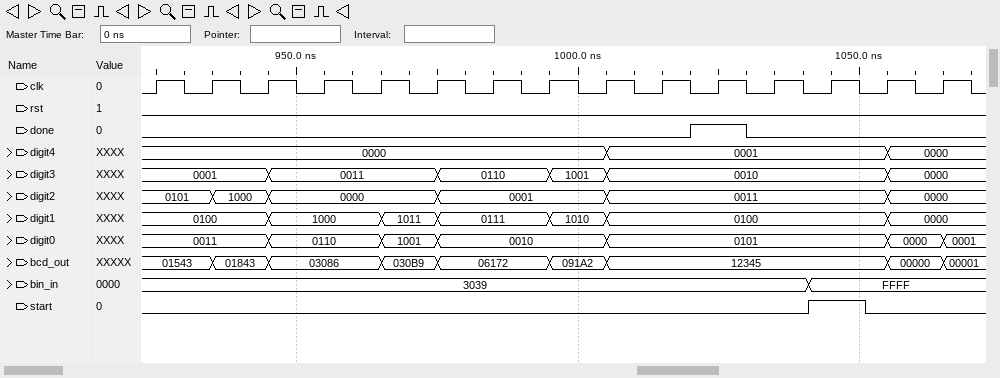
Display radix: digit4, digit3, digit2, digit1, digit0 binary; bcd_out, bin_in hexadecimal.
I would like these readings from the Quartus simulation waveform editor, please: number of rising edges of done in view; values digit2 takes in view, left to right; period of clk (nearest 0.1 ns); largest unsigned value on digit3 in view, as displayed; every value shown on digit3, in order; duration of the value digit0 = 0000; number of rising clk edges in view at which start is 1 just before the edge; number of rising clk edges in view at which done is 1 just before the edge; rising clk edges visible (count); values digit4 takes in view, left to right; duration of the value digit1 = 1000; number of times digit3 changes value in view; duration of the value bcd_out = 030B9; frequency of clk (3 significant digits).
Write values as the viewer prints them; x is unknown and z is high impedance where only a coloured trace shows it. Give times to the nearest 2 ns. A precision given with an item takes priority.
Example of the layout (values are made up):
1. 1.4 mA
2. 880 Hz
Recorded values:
1. 1
2. 0101, 1000, 0000, 0001, 0011, 0000
3. 10 ns
4. 1001
5. 0001, 0011, 0110, 1001, 0010, 0000
6. 10 ns
7. 1
8. 1
9. 15
10. 0000, 0001, 0000
11. 20 ns
12. 5
13. 10 ns
14. 100 MHz
